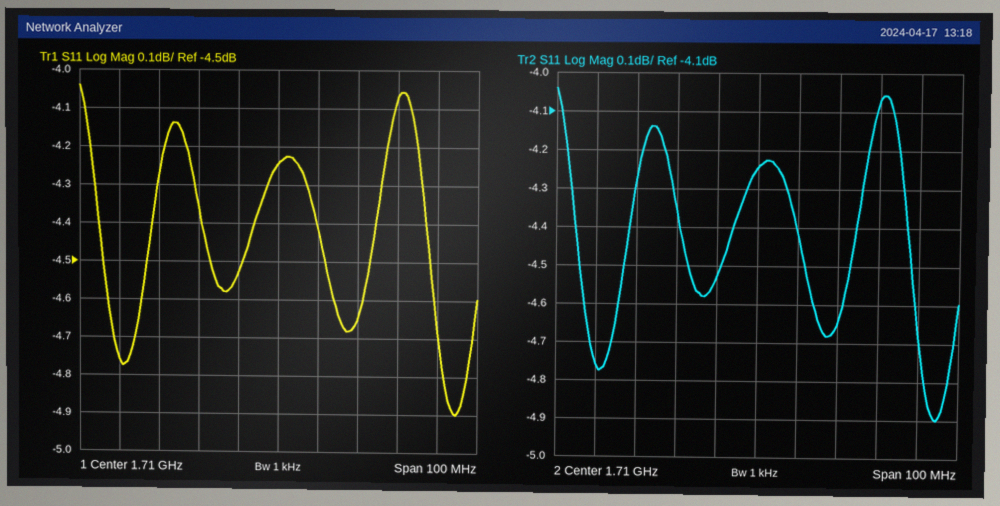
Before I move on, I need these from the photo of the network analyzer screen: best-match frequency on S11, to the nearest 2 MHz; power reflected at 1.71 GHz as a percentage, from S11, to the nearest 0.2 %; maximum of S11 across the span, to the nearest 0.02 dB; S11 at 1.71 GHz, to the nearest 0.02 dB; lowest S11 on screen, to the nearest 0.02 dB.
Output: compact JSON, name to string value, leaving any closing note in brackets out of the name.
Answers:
{"best-match frequency on S11, to the nearest 2 MHz": "1.754 GHz", "power reflected at 1.71 GHz as a percentage, from S11, to the nearest 0.2 %": "37.6 %", "maximum of S11 across the span, to the nearest 0.02 dB": "-4.04 dB", "S11 at 1.71 GHz, to the nearest 0.02 dB": "-4.24 dB", "lowest S11 on screen, to the nearest 0.02 dB": "-4.90 dB"}
